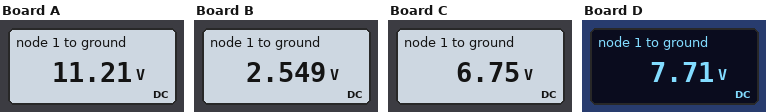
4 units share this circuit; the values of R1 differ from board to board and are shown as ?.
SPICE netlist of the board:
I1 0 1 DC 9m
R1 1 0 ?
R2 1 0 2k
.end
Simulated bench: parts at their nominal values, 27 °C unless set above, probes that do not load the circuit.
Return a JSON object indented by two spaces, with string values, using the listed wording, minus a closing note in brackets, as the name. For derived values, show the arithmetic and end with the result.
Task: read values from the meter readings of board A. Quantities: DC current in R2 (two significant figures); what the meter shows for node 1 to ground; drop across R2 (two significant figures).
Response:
{
  "DC current in R2": "(11.21 V) / 2 kΩ = 5.6 mA",
  "what the meter shows for node 1 to ground": "11.21 V",
  "drop across R2": "11.21 V = 11 V"
}
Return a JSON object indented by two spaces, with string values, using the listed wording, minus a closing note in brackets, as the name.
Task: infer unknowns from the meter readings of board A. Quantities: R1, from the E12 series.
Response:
{
  "R1, from the E12 series": "3.3 kΩ"
}
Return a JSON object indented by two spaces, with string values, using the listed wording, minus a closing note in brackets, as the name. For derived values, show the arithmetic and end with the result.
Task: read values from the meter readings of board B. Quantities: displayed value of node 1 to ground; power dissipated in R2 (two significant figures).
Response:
{
  "displayed value of node 1 to ground": "2.549 V",
  "power dissipated in R2": "(2.549 V)^2 / 2 kΩ = 3.2 mW"
}
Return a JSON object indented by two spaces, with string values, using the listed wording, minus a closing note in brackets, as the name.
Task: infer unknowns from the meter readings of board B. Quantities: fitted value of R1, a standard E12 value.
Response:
{
  "fitted value of R1, a standard E12 value": "330 Ω"
}
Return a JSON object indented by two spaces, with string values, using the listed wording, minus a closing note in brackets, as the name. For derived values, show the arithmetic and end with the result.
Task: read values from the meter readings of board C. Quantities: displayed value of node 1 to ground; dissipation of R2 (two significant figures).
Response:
{
  "displayed value of node 1 to ground": "6.75 V",
  "dissipation of R2": "(6.75 V)^2 / 2 kΩ = 23 mW"
}
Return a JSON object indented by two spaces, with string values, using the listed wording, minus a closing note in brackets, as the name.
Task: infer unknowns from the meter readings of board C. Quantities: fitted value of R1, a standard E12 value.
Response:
{
  "fitted value of R1, a standard E12 value": "1.2 kΩ"
}
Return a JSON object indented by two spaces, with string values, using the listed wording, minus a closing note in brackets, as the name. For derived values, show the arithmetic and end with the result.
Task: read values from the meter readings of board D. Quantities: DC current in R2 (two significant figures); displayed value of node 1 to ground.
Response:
{
  "DC current in R2": "(7.71 V) / 2 kΩ = 3.9 mA",
  "displayed value of node 1 to ground": "7.71 V"
}
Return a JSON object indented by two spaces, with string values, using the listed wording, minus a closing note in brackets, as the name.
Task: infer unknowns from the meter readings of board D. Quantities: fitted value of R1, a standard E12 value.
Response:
{
  "fitted value of R1, a standard E12 value": "1.5 kΩ"
}
